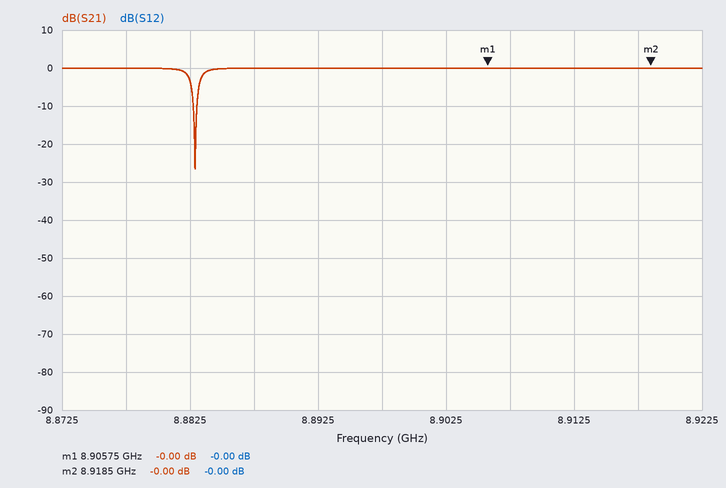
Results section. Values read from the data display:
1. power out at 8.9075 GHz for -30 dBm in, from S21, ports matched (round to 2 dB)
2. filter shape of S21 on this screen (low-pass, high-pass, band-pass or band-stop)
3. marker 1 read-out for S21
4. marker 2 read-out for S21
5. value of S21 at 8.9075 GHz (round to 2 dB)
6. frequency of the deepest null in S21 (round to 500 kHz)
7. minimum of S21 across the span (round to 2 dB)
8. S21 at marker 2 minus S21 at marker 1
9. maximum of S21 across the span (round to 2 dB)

-30 dBm
band-stop
-0.00 dB
-0.00 dB
0 dB
8.8830 GHz
-26 dB
0.00 dB
0 dB
